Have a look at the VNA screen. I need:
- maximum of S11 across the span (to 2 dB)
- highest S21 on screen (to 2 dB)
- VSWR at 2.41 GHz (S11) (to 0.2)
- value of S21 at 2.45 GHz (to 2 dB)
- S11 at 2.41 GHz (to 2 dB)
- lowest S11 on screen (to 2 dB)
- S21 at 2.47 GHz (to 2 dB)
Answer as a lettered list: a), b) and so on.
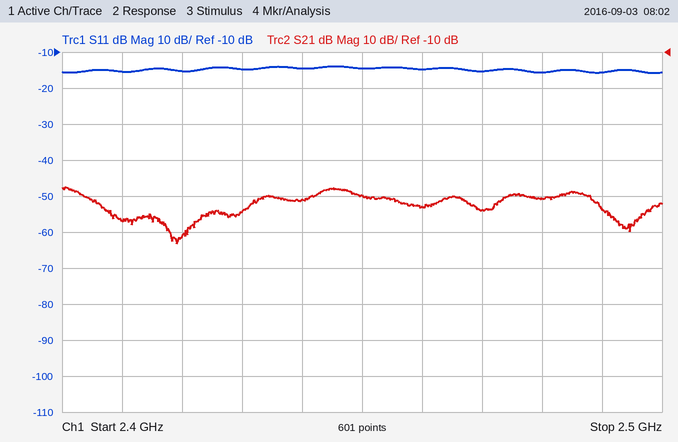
a) -14 dB
b) -48 dB
c) 1.4
d) -50 dB
e) -16 dB
f) -16 dB
g) -54 dB
